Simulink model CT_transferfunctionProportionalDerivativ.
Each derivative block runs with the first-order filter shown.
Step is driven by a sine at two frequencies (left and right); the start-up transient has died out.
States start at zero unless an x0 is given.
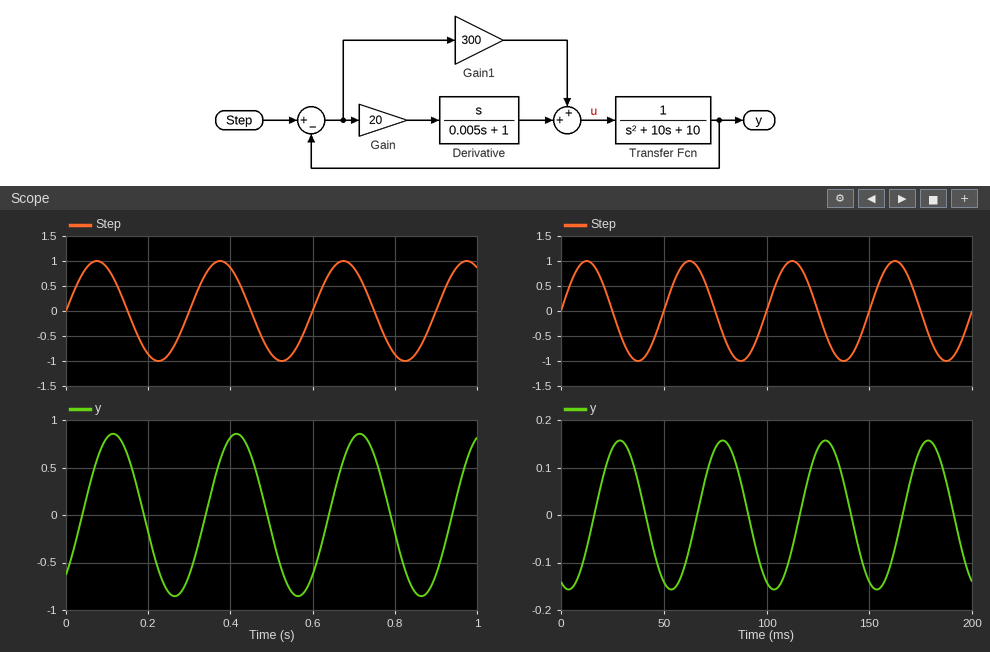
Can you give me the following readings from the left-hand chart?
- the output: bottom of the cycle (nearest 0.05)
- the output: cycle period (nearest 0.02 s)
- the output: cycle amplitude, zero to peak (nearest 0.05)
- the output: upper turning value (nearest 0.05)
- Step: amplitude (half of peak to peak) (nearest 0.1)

-0.85
0.30 s
0.85
0.85
1.0
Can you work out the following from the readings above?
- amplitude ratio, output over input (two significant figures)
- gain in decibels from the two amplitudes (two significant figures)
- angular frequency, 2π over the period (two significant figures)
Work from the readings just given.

0.85
-1.4 dB
21 rad/s
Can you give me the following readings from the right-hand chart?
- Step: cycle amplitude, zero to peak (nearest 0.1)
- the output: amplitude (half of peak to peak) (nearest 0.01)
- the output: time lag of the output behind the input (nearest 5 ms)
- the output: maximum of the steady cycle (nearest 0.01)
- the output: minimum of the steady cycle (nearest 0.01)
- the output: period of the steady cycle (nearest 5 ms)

1.0
0.16
15 ms
0.16
-0.16
50 ms
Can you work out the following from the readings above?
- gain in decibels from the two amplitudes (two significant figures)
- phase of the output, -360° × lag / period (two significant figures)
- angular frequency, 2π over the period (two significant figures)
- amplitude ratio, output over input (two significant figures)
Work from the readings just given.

-16 dB
-110°
0.13 rad/ms
0.16
